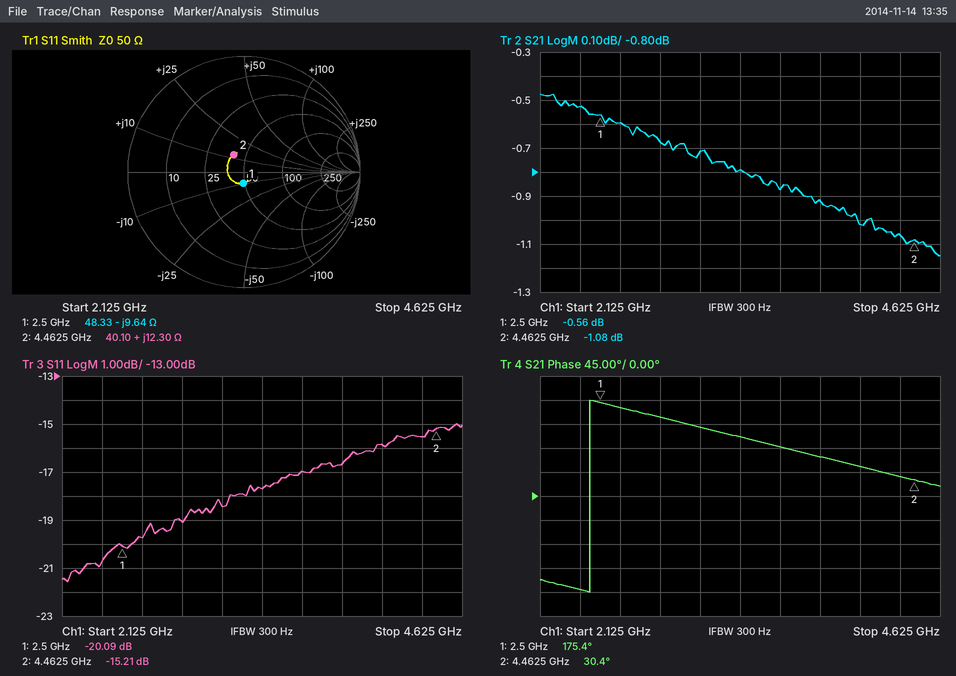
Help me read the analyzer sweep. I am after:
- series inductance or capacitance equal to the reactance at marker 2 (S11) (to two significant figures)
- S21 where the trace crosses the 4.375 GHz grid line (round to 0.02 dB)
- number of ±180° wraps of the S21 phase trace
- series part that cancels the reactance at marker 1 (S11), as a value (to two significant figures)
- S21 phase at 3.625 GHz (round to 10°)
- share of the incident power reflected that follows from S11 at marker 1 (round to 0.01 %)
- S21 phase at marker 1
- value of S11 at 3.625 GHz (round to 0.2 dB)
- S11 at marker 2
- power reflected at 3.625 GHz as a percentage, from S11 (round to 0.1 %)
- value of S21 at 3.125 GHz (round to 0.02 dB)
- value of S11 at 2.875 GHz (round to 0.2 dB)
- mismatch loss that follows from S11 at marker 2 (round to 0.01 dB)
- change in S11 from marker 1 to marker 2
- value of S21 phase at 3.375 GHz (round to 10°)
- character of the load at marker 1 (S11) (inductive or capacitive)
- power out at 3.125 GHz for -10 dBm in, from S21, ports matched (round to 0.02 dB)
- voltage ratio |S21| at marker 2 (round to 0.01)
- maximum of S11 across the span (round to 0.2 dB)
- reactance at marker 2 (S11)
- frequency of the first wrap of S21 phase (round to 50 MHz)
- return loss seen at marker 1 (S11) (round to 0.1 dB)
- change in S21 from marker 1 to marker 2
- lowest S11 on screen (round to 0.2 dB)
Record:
440 pH
-1.06 dB
1
610 pH
90°
0.98 %
175.4°
-17.0 dB
-15.21 dB
2.0 %
-0.72 dB
-19.0 dB
0.13 dB
4.88 dB
110°
capacitive
-10.72 dBm
0.88
-15.0 dB
+12.30 Ω
2.45 GHz
20.1 dB
-0.52 dB
-21.6 dB
